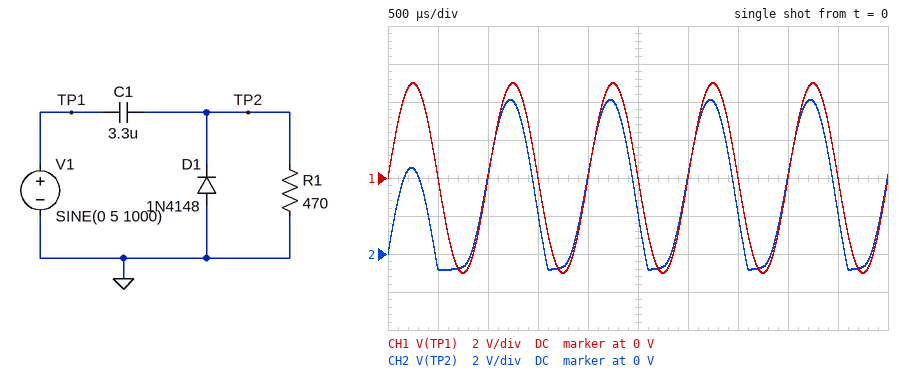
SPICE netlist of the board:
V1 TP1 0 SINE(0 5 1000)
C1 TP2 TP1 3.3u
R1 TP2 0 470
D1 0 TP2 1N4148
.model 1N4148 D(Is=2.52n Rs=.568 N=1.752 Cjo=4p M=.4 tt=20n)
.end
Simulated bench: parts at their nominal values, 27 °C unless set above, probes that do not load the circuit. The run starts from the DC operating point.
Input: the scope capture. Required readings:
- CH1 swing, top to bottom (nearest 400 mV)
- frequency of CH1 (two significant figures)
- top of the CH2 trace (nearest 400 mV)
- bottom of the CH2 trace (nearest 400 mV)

10.0 V
1.0 kHz
8.0 V
-800 mV
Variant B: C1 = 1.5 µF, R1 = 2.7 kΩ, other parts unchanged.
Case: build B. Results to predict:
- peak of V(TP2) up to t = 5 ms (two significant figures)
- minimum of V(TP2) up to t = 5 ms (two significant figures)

8.9 V
-780 mV
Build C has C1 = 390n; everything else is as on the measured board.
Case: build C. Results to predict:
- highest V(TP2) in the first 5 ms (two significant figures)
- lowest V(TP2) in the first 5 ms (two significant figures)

4.1 V
-700 mV
